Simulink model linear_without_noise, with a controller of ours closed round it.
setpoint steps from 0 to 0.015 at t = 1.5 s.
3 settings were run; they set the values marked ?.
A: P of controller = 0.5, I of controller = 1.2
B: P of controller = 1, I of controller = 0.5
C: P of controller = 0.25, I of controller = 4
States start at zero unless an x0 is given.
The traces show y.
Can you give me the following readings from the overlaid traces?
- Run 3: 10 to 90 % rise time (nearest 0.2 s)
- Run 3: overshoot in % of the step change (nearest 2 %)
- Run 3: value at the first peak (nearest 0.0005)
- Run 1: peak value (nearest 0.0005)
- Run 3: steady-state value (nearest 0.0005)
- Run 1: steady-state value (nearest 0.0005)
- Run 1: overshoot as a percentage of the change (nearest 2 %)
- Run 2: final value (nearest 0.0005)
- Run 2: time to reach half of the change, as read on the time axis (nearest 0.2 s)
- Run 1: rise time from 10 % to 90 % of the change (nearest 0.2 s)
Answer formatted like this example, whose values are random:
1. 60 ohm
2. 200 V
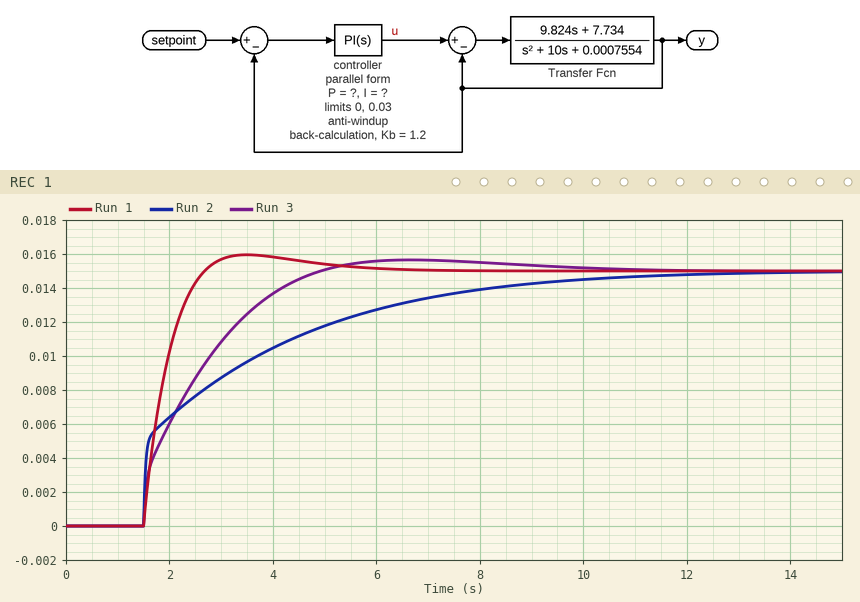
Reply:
1. 2.4 s
2. 4 %
3. 0.0155
4. 0.0160
5. 0.0150
6. 0.0150
7. 6 %
8. 0.0150
9. 2.4 s
10. 0.8 s
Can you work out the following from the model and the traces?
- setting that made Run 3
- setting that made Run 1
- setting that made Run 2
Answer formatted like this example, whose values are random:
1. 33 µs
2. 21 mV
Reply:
1. A
2. C
3. B
